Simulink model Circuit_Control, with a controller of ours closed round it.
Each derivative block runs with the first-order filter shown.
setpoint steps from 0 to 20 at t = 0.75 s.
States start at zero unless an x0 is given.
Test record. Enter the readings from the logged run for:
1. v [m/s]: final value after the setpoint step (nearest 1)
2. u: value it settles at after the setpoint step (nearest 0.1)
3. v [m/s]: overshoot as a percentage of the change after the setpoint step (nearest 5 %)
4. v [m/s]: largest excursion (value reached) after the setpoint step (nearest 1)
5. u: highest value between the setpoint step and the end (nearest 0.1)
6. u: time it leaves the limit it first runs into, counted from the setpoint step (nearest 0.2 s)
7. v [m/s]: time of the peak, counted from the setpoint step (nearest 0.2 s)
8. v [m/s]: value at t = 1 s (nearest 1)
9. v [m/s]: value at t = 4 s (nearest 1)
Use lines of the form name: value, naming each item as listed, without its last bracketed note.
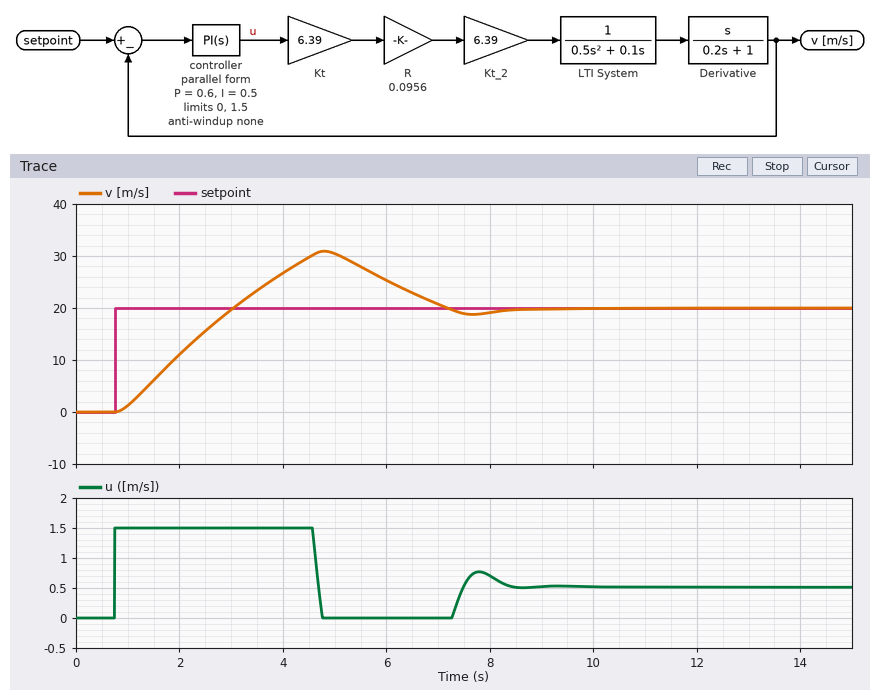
v [m/s]: final value after the setpoint step: 20
u: value it settles at after the setpoint step: 0.5
v [m/s]: overshoot as a percentage of the change after the setpoint step: 55 %
v [m/s]: largest excursion (value reached) after the setpoint step: 31
u: highest value between the setpoint step and the end: 1.5
u: time it leaves the limit it first runs into, counted from the setpoint step: 3.8 s
v [m/s]: time of the peak, counted from the setpoint step: 4.0 s
v [m/s]: value at t = 1 s: 1
v [m/s]: value at t = 4 s: 27
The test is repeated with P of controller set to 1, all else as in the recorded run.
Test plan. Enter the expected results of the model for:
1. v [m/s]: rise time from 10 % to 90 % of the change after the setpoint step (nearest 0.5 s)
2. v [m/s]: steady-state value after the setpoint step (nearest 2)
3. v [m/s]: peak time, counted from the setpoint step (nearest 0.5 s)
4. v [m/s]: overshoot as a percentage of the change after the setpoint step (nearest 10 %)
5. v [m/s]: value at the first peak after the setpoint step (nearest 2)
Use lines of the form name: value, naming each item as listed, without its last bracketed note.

v [m/s]: rise time from 10 % to 90 % of the change after the setpoint step: 1.5 s
v [m/s]: steady-state value after the setpoint step: 20
v [m/s]: peak time, counted from the setpoint step: 3.5 s
v [m/s]: overshoot as a percentage of the change after the setpoint step: 40 %
v [m/s]: value at the first peak after the setpoint step: 28
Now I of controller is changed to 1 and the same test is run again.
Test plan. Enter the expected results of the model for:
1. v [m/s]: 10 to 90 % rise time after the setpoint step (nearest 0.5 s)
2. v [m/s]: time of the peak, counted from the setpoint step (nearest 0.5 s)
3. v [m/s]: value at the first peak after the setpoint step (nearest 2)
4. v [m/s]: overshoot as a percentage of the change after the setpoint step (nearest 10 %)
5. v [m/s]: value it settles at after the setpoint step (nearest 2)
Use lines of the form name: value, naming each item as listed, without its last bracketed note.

v [m/s]: 10 to 90 % rise time after the setpoint step: 1.5 s
v [m/s]: time of the peak, counted from the setpoint step: 4.5 s
v [m/s]: value at the first peak after the setpoint step: 34
v [m/s]: overshoot as a percentage of the change after the setpoint step: 70 %
v [m/s]: value it settles at after the setpoint step: 20
